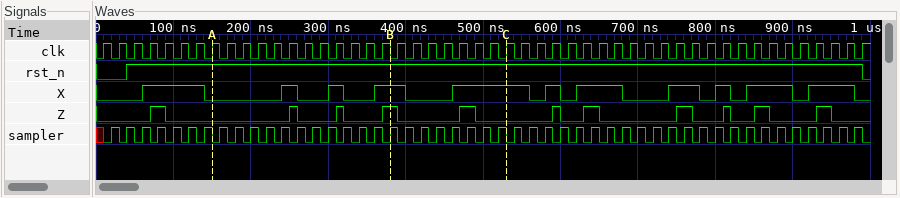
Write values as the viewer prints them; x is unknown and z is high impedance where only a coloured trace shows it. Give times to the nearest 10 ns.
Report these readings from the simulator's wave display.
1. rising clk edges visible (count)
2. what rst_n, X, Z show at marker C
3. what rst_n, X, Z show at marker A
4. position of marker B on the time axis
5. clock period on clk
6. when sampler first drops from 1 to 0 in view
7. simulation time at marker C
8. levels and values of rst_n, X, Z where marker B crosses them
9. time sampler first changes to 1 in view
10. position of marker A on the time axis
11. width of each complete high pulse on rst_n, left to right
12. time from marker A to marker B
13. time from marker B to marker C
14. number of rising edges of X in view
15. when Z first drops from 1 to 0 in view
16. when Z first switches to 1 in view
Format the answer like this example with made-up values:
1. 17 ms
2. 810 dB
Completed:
1. 50
2. rst_n=1, X=1, Z=0
3. rst_n=1, X=0, Z=0
4. 380 ns
5. 20 ns
6. 30 ns
7. 530 ns
8. rst_n=1, X=1, Z=1
9. 20 ns
10. 150 ns
11. 950 ns
12. 230 ns
13. 150 ns
14. 11
15. 90 ns
16. 70 ns
